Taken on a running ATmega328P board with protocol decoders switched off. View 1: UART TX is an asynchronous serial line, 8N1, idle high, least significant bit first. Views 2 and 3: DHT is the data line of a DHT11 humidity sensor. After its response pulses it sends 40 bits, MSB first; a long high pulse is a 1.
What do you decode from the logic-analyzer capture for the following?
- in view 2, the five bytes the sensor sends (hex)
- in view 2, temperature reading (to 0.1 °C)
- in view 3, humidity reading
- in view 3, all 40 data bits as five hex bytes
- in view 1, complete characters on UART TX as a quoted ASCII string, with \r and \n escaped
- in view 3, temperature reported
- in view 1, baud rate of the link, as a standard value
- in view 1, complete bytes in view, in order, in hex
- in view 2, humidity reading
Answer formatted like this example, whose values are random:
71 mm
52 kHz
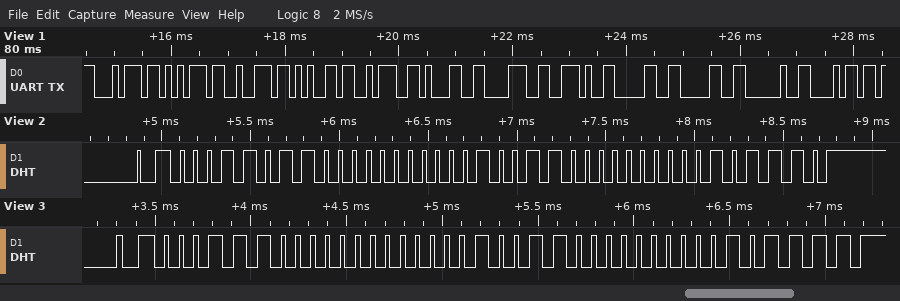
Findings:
1B 00 13 00 2E
19.0 °C
28 %
1C 00 13 00 2F
"ture:18.00 h"
19.0 °C
9600 baud
74 75 72 65 3A 31 38 2E 30 30 20 68
27 %
